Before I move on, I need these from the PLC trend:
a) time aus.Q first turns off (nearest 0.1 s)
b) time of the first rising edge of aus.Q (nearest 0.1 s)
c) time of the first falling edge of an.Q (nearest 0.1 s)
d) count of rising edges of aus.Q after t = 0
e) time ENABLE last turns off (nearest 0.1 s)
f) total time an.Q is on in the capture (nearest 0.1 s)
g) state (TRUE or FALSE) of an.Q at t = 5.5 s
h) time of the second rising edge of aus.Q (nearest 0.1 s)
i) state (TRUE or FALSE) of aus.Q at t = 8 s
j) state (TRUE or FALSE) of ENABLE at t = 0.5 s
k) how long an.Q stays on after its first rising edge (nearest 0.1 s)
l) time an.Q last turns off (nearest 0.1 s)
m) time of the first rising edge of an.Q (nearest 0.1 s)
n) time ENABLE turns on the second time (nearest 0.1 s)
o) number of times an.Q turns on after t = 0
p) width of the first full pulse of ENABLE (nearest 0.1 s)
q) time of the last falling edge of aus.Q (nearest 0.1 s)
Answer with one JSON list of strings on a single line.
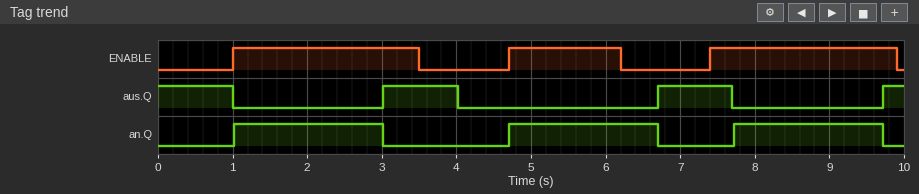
["1.0 s", "3.0 s", "3.0 s", "3", "9.9 s", "6.0 s", "TRUE", "6.7 s", "FALSE", "FALSE", "2.0 s", "9.7 s", "1.0 s", "4.7 s", "3", "2.5 s", "7.7 s"]
